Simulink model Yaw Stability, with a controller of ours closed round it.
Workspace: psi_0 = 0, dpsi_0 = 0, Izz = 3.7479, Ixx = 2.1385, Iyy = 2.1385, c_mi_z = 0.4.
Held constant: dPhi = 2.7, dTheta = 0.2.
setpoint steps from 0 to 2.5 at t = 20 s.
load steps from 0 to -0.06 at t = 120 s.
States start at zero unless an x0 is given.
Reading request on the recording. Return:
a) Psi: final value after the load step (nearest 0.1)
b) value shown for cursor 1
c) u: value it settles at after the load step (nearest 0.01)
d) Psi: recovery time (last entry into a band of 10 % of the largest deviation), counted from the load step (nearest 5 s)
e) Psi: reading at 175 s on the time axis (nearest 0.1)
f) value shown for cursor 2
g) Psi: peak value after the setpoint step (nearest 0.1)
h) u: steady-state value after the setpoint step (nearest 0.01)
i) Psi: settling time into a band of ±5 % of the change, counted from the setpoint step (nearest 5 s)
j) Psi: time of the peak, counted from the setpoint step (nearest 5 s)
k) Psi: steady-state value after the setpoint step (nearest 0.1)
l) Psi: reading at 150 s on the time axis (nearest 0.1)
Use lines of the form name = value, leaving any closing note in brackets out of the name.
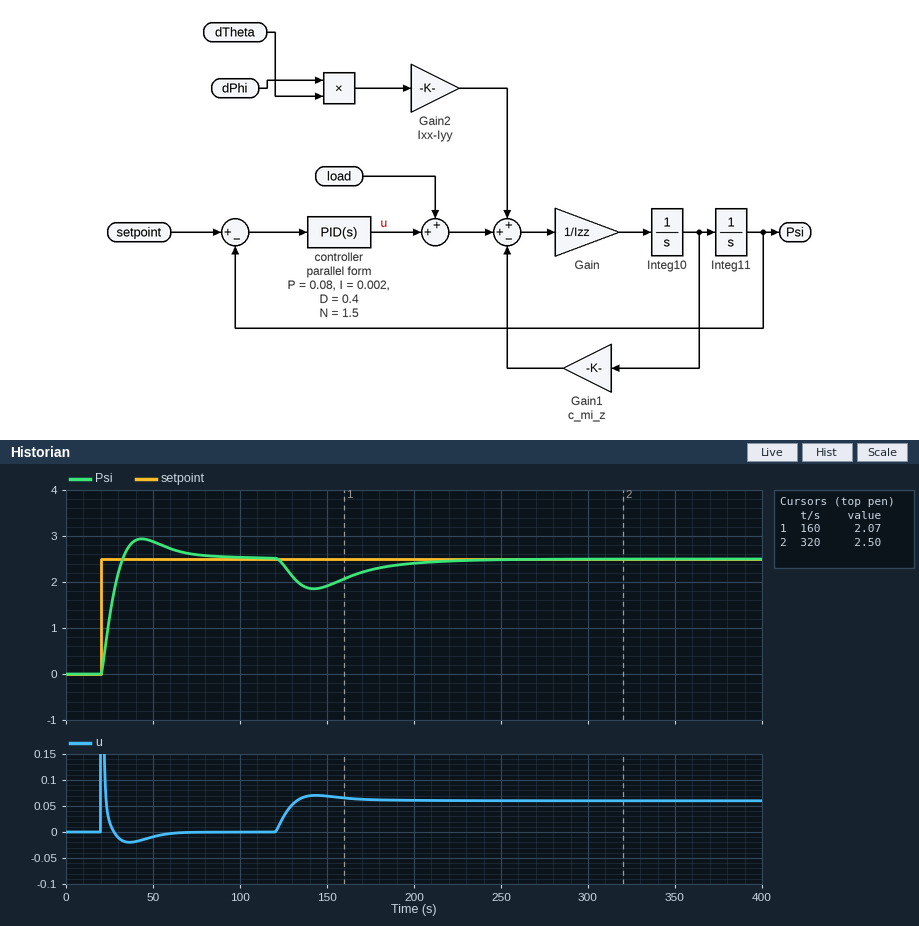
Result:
Psi: final value after the load step = 2.5
value shown for cursor 1 = 2.07
u: value it settles at after the load step = 0.06
Psi: recovery time (last entry into a band of 10 % of the largest deviation), counted from the load step = 90 s
Psi: reading at 175 s on the time axis = 2.3
value shown for cursor 2 = 2.50
Psi: peak value after the setpoint step = 2.9
u: steady-state value after the setpoint step = 0.00
Psi: settling time into a band of ±5 % of the change, counted from the setpoint step = 50 s
Psi: time of the peak, counted from the setpoint step = 25 s
Psi: steady-state value after the setpoint step = 2.5
Psi: reading at 150 s on the time axis = 1.9
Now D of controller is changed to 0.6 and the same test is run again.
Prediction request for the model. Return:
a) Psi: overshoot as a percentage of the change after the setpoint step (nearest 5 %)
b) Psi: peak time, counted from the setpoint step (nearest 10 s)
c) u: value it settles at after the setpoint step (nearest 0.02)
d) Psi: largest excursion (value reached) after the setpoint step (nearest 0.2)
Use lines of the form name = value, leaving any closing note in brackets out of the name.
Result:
Psi: overshoot as a percentage of the change after the setpoint step = 10 %
Psi: peak time, counted from the setpoint step = 30 s
u: value it settles at after the setpoint step = 0.00
Psi: largest excursion (value reached) after the setpoint step = 2.8
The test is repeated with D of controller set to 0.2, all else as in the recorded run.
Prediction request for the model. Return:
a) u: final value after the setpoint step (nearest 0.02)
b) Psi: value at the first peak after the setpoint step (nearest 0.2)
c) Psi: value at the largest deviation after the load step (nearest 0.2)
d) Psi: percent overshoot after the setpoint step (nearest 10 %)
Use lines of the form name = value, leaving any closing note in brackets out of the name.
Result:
u: final value after the setpoint step = 0.00
Psi: value at the first peak after the setpoint step = 3.2
Psi: value at the largest deviation after the load step = 1.8
Psi: percent overshoot after the setpoint step = 30 %
